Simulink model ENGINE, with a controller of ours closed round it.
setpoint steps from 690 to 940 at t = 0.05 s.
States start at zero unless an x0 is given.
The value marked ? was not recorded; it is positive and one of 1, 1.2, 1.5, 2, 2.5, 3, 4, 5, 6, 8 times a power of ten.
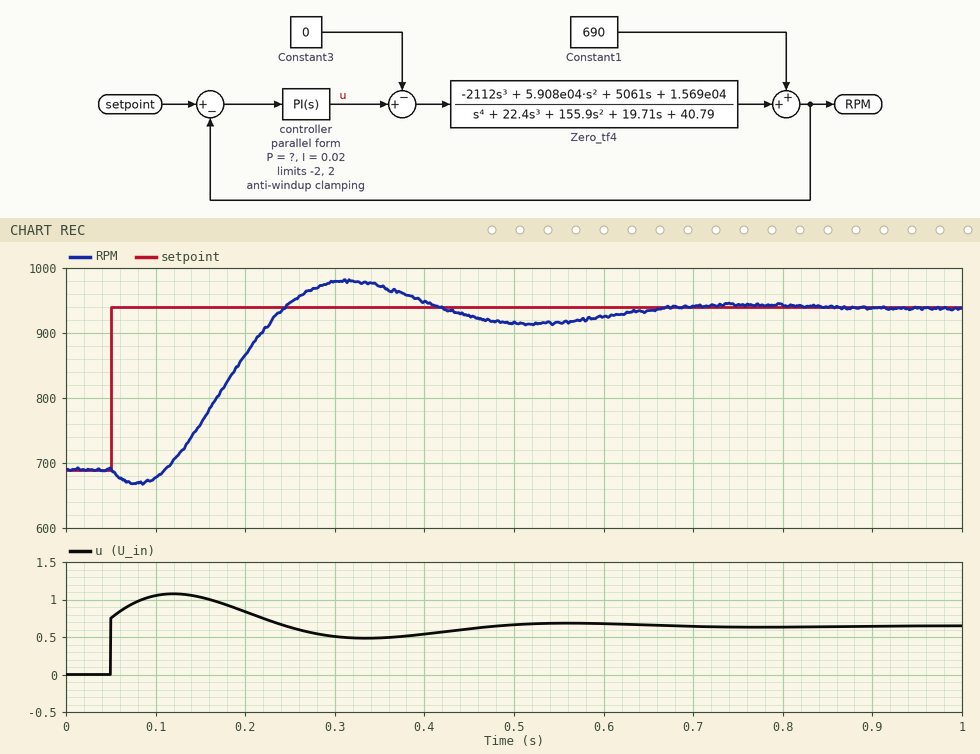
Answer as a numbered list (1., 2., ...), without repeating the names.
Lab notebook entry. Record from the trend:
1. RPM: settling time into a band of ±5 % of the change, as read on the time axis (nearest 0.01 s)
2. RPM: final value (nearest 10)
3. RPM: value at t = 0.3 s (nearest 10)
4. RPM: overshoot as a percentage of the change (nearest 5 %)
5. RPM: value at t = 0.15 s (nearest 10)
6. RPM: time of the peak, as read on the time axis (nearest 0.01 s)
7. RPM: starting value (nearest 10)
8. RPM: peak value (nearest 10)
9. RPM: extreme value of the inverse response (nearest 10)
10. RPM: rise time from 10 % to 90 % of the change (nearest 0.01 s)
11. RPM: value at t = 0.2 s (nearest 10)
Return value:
1. 0.61 s
2. 940
3. 980
4. 15 %
5. 760
6. 0.31 s
7. 690
8. 980
9. 670
10. 0.10 s
11. 870
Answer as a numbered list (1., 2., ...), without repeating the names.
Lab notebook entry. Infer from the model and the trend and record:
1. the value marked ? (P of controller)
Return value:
1. 0.003
